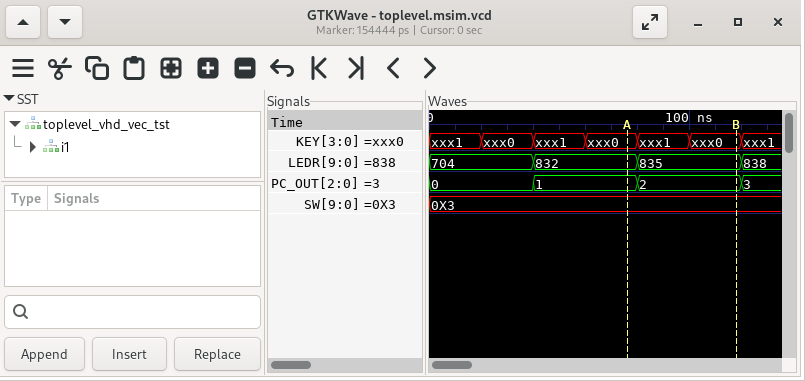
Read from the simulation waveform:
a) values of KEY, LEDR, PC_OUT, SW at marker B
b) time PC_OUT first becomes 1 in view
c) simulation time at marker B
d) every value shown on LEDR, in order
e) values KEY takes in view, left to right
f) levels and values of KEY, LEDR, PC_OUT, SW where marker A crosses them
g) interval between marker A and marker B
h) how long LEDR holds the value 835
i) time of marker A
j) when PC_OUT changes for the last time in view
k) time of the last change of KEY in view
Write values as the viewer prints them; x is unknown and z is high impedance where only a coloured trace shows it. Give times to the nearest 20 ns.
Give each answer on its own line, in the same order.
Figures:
KEY=xxx0, LEDR=835, PC_OUT=2, SW=0X3
40 ns
120 ns
704, 832, 835, 838
xxx1, xxx0, xxx1, xxx0, xxx1, xxx0, xxx1
KEY=xxx0, LEDR=832, PC_OUT=1, SW=0X3
40 ns
40 ns
80 ns
120 ns
120 ns
